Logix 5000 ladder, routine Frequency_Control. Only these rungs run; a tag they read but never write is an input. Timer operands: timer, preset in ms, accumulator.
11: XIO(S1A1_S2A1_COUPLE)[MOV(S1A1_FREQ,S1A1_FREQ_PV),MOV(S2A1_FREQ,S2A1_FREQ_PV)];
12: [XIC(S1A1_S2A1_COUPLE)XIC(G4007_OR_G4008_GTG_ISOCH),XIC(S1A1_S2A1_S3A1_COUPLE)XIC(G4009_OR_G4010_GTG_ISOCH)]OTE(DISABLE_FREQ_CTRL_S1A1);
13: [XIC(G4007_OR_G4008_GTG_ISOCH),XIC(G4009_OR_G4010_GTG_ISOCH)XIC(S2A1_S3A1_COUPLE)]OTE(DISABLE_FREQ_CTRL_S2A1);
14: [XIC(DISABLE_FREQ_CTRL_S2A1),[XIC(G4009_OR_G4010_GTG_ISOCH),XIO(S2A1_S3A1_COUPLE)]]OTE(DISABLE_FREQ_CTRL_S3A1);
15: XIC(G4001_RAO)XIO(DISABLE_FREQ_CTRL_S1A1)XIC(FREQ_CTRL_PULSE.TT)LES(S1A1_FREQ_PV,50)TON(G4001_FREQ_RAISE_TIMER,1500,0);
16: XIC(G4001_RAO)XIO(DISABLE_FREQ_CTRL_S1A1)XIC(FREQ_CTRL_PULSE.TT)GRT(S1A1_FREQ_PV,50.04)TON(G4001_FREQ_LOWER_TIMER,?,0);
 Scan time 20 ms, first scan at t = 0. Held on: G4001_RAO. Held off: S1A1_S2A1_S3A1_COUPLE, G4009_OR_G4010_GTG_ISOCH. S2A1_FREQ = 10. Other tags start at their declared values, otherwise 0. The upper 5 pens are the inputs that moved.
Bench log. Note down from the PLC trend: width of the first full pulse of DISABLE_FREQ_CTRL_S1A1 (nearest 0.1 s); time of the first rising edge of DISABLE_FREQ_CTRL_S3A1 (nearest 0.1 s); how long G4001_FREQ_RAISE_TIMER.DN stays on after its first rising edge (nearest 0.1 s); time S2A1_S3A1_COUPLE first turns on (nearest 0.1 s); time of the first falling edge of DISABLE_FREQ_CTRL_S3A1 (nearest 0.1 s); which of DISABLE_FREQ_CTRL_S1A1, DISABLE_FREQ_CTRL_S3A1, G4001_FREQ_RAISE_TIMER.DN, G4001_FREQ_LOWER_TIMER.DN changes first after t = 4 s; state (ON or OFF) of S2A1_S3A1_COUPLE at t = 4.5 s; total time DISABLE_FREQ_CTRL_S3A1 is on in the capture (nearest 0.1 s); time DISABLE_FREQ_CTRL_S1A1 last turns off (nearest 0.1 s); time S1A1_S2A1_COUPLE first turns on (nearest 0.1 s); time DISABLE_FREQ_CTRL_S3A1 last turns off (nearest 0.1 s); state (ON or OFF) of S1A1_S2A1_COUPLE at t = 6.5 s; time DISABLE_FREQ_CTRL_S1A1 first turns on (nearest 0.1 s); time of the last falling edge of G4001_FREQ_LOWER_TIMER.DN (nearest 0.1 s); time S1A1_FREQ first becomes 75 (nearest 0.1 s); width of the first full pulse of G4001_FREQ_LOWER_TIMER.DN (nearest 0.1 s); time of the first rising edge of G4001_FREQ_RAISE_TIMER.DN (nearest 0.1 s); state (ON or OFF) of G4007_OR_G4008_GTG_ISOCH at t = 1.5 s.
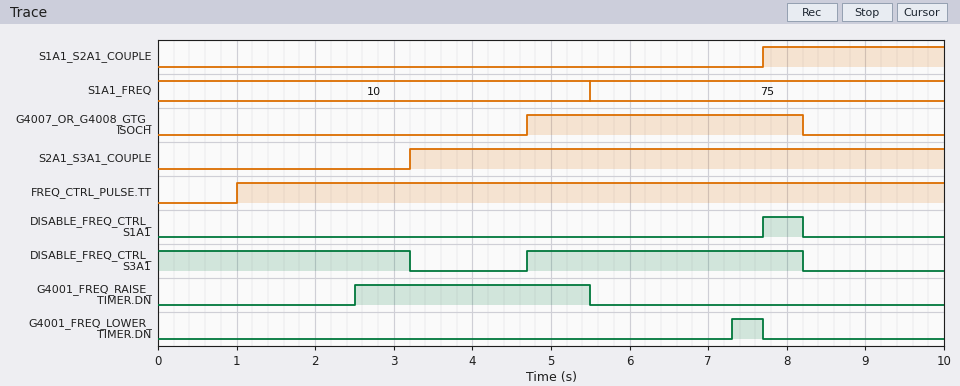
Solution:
0.5 s
4.7 s
3.0 s
3.2 s
3.2 s
DISABLE_FREQ_CTRL_S3A1
ON
6.7 s
8.2 s
7.7 s
8.2 s
OFF
7.7 s
7.7 s
5.5 s
0.4 s
2.5 s
OFF
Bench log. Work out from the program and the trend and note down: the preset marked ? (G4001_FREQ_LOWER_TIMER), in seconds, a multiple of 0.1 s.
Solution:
1.8 s
